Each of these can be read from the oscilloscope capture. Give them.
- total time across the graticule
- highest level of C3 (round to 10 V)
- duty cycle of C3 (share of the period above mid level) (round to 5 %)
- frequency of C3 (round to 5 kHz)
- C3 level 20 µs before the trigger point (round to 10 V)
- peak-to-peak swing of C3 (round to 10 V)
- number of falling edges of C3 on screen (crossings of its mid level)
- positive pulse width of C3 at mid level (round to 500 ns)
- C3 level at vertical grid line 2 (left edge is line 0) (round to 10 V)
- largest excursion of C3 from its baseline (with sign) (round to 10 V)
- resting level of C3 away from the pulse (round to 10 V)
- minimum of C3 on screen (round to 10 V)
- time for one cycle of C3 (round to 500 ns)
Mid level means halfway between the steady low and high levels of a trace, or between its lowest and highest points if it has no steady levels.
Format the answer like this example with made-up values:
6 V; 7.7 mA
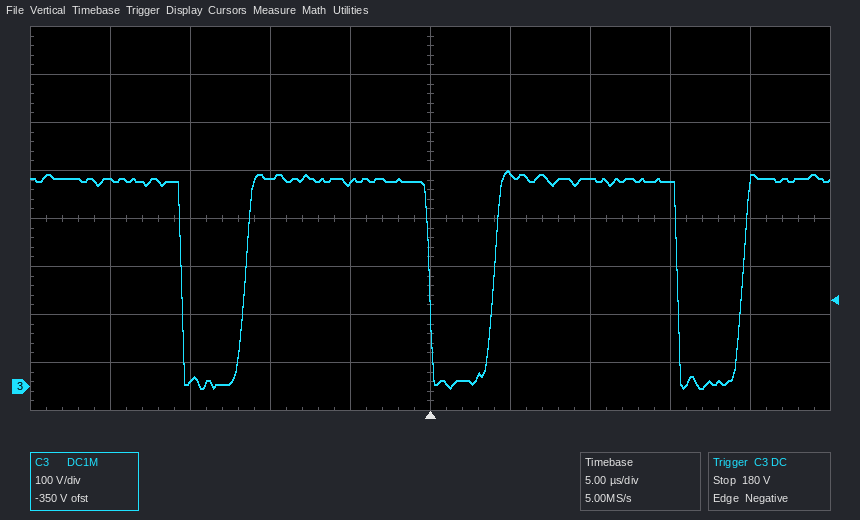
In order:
50 µs; 450 V; 75 %; 65 kHz; 430 V; 450 V; 3; 11.5 µs; 10 V; -430 V; 430 V; 0 V; 15.5 µs
